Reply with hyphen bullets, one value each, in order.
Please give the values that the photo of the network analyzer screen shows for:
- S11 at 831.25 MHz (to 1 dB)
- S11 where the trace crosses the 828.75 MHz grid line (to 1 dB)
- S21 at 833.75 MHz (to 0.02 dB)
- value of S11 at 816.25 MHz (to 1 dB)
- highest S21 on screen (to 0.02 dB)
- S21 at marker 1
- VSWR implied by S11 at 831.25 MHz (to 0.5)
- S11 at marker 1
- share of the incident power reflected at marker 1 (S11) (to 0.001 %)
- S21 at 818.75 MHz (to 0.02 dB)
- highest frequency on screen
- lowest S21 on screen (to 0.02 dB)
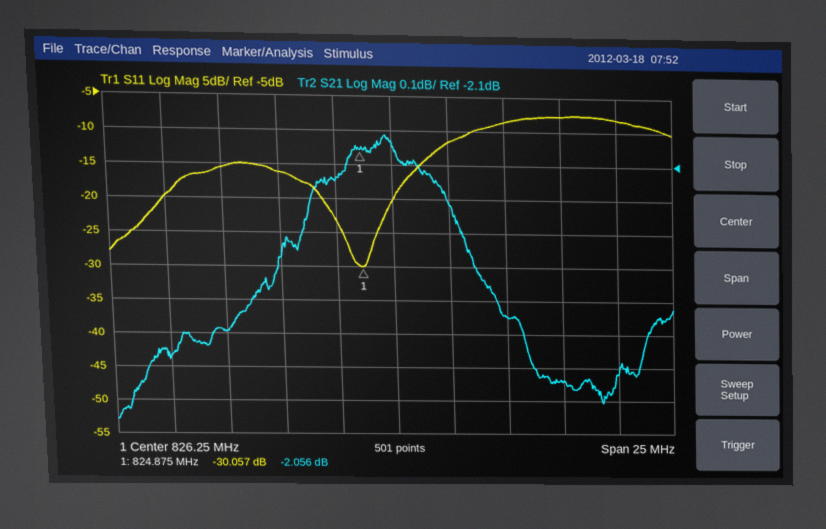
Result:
- -9 dB
- -12 dB
- -2.74 dB
- -20 dB
- -2.02 dB
- -2.056 dB
- 2.0
- -30.057 dB
- 0.099 %
- -2.60 dB
- 838.75 MHz
- -2.86 dB
